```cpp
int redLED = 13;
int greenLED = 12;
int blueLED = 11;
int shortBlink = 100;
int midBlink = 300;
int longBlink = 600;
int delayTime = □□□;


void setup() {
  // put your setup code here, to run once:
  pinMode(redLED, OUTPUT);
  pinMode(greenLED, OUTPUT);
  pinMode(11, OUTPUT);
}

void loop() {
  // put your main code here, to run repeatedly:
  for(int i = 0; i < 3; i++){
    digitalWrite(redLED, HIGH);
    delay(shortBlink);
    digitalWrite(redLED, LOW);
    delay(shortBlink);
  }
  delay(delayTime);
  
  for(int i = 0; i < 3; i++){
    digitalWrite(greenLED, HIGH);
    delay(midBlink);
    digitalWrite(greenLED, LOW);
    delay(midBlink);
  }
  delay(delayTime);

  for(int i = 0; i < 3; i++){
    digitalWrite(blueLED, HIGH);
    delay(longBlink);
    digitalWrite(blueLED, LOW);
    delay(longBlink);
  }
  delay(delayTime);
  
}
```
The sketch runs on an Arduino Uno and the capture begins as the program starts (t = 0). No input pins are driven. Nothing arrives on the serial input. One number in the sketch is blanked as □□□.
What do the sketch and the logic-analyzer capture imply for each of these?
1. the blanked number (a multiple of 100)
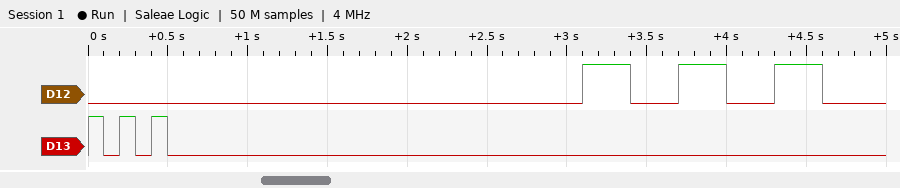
2500
